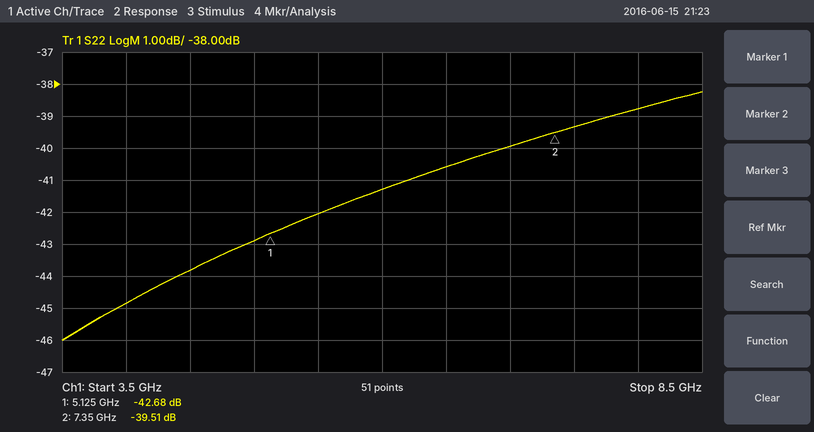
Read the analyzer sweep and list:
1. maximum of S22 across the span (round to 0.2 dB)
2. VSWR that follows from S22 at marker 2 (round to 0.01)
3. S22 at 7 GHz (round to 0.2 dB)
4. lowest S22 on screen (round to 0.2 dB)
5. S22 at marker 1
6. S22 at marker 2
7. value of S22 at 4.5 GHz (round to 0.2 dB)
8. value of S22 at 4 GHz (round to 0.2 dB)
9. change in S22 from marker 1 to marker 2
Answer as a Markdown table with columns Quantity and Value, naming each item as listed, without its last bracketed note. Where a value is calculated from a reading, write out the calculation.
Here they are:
| Quantity | Value |
|---|---|
| maximum of S22 across the span | -38.2 dB |
| VSWR that follows from S22 at marker 2 | (1 + 0.0106)/(1 − 0.0106) ≈ 1.02 |
| S22 at 7 GHz | -40.0 dB |
| lowest S22 on screen | -46.0 dB |
| S22 at marker 1 | -42.68 dB |
| S22 at marker 2 | -39.51 dB |
| value of S22 at 4.5 GHz | -43.8 dB |
| value of S22 at 4 GHz | -44.8 dB |
| change in S22 from marker 1 to marker 2 | -39.51 − (-42.68) = 3.17 dB |
